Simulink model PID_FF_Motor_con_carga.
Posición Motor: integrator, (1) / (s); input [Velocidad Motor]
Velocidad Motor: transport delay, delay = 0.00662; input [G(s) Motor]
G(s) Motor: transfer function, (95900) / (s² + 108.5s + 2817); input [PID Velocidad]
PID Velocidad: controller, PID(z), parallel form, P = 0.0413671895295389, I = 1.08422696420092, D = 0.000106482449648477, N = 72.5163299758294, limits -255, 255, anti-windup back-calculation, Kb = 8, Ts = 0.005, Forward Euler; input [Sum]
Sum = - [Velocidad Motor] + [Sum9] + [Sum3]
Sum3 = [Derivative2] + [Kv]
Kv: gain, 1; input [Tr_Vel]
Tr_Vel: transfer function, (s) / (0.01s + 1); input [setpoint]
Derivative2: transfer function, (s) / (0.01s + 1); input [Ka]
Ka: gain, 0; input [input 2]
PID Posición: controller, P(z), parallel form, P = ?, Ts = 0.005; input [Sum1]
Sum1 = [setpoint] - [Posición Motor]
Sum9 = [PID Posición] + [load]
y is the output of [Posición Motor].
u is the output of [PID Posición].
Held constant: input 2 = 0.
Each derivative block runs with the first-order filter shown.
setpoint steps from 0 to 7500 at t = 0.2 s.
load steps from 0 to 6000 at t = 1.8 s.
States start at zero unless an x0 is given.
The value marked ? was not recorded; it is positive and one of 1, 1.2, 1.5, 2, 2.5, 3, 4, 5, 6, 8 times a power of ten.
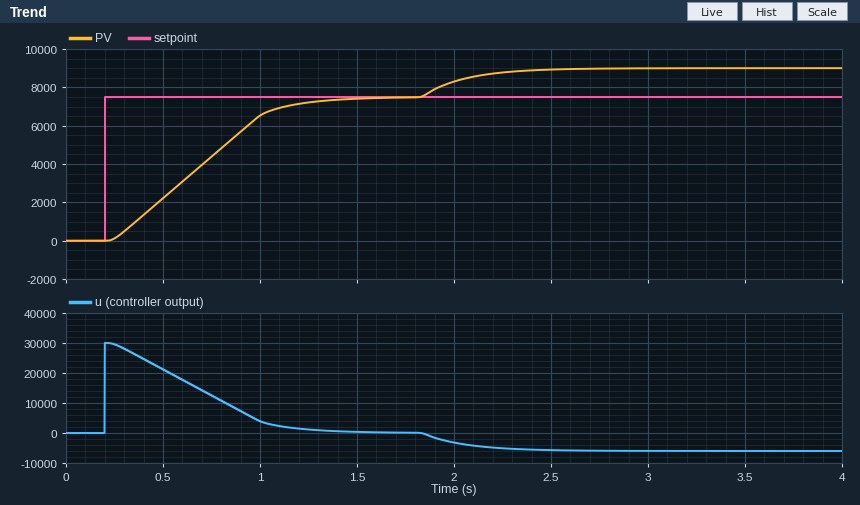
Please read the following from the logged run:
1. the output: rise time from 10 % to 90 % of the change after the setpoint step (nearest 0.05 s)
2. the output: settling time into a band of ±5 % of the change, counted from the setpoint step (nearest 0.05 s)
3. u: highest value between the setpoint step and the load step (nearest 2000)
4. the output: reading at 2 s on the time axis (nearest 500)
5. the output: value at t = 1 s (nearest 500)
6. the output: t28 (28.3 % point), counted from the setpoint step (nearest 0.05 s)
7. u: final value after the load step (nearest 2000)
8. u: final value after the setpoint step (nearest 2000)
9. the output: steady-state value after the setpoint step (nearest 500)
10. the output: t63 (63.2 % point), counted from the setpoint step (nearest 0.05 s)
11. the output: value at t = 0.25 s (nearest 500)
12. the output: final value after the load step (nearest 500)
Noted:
0.70 s
1.00 s
30000
8500
6500
0.30 s
-6000
0
7500
0.60 s
0
9000
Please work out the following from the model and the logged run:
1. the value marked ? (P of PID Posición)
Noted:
4
